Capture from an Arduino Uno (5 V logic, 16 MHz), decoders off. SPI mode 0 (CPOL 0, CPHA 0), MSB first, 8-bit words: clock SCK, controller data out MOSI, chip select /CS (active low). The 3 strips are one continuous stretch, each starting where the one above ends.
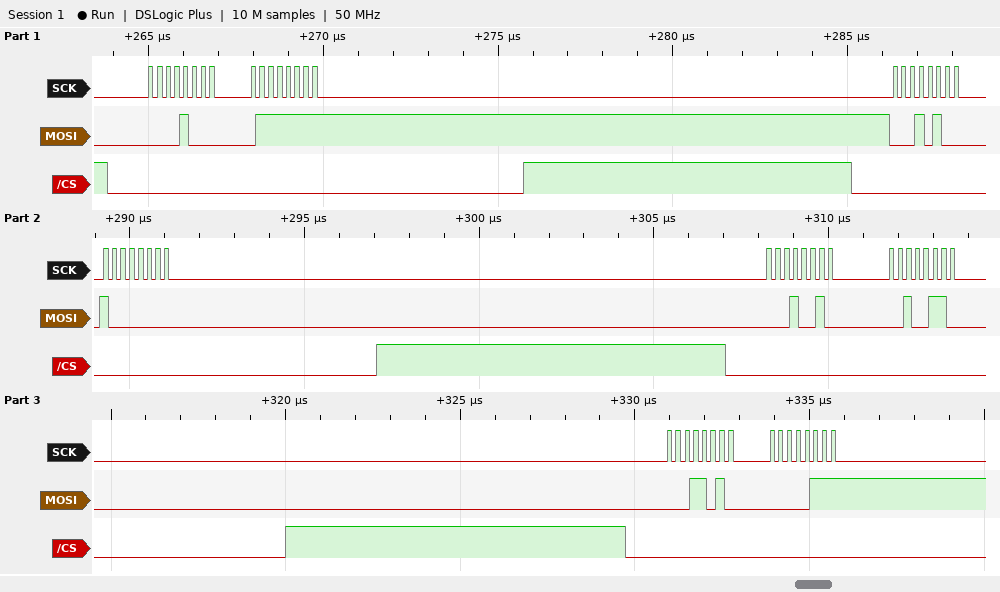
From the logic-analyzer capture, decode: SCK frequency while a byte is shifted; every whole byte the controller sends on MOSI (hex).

4 MHz
08 7F 14 80 12 26 1A 07
